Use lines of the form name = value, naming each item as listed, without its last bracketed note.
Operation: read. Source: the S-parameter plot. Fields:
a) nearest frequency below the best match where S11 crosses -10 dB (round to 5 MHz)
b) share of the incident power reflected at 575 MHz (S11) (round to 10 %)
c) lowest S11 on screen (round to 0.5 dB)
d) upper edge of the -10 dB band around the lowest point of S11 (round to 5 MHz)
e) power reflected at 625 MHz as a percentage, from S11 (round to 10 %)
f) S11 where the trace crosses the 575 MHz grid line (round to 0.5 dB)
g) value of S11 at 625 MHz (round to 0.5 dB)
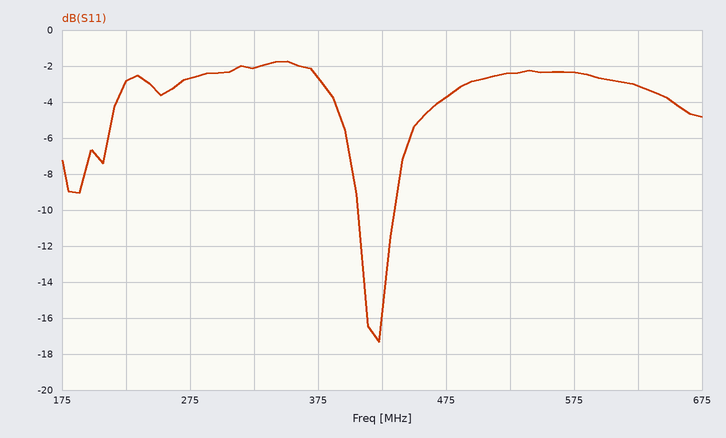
nearest frequency below the best match where S11 crosses -10 dB = 405 MHz
share of the incident power reflected at 575 MHz (S11) = 60 %
lowest S11 on screen = -17.5 dB
upper edge of the -10 dB band around the lowest point of S11 = 435 MHz
power reflected at 625 MHz as a percentage, from S11 = 50 %
S11 where the trace crosses the 575 MHz grid line = -2.5 dB
value of S11 at 625 MHz = -3.0 dB
